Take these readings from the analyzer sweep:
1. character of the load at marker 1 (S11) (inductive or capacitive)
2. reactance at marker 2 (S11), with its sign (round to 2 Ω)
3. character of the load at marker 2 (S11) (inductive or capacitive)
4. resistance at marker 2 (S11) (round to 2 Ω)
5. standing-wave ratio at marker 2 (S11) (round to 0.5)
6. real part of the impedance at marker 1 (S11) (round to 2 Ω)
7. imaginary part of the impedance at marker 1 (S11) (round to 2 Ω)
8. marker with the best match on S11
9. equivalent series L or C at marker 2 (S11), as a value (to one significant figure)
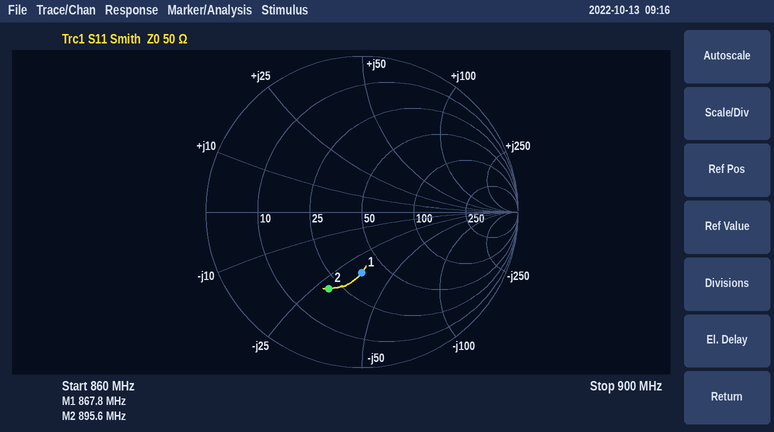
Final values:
capacitive
-28 Ω
capacitive
20 Ω
3.5
36 Ω
-34 Ω
marker 1
6 pF
